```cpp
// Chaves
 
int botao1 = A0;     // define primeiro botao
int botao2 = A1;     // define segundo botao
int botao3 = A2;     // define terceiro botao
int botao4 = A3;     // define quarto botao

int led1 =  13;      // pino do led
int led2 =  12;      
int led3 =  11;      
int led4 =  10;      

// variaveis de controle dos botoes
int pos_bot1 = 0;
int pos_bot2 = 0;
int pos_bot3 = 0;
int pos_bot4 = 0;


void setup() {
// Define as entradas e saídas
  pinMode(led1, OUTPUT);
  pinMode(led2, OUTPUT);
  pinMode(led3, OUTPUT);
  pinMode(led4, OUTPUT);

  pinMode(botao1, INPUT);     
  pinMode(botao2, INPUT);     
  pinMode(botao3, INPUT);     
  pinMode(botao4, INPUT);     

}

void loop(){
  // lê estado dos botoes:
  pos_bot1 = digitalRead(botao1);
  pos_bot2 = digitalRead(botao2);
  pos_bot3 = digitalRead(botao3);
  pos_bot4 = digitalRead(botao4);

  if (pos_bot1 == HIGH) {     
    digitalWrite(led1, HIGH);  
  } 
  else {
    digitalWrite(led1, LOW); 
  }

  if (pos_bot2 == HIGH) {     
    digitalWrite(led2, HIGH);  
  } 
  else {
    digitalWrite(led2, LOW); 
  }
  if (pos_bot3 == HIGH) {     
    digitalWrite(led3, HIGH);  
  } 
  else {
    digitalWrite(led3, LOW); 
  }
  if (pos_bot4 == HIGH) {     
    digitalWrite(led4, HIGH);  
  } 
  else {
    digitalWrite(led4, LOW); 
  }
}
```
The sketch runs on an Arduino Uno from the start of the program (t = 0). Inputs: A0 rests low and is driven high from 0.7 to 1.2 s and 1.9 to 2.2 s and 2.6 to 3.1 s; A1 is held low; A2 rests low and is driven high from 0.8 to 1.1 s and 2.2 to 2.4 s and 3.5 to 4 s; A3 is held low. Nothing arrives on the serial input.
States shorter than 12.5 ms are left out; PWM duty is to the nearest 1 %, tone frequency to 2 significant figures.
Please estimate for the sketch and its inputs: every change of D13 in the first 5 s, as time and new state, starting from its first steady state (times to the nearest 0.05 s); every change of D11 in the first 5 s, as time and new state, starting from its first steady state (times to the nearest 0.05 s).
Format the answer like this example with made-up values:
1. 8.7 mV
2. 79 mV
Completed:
1. 0 s low; 0.7 s high; 1.2 s low; 1.9 s high; 2.2 s low; 2.6 s high; 3.1 s low
2. 0 s low; 0.8 s high; 1.1 s low; 2.2 s high; 2.4 s low; 3.5 s high; 4 s low
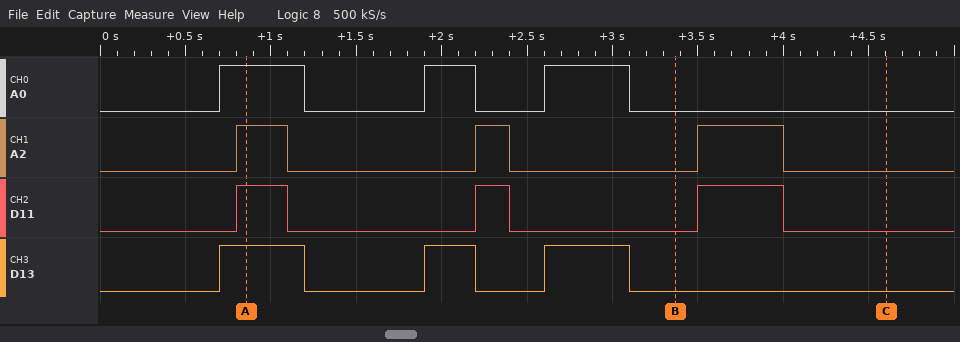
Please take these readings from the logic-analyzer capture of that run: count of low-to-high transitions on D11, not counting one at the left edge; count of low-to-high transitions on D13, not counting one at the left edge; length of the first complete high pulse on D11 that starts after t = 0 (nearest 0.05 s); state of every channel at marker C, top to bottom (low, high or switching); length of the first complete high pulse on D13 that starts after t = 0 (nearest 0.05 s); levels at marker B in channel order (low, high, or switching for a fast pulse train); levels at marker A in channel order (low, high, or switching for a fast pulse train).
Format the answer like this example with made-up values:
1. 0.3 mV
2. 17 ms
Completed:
1. 3
2. 3
3. 0.30 s
4. A0 low, A2 low, D11 low, D13 low
5. 0.50 s
6. A0 low, A2 low, D11 low, D13 low
7. A0 high, A2 high, D11 high, D13 high
